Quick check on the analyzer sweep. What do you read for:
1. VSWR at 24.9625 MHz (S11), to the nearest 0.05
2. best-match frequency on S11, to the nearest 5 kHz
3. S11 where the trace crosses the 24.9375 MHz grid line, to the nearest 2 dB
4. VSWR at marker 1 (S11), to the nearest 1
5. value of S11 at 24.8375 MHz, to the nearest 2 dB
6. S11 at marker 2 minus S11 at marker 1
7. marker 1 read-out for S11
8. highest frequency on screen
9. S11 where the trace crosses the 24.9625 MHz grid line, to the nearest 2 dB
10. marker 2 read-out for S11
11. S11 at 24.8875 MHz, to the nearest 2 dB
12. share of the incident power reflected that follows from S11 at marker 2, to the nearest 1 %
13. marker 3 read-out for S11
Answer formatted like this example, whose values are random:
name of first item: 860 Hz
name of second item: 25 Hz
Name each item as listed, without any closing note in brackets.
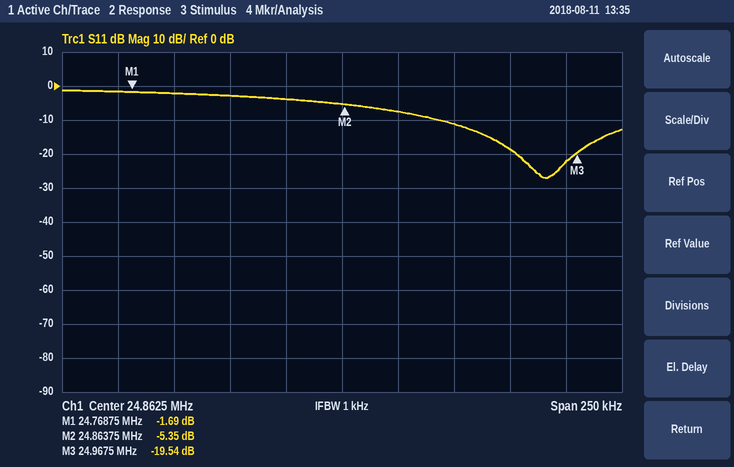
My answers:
VSWR at 24.9625 MHz (S11), to the nearest 0.05: 1.15
best-match frequency on S11, to the nearest 5 kHz: 24.955 MHz
S11 where the trace crosses the 24.9375 MHz grid line, to the nearest 2 dB: -18 dB
VSWR at marker 1 (S11), to the nearest 1: 10
value of S11 at 24.8375 MHz, to the nearest 2 dB: -4 dB
S11 at marker 2 minus S11 at marker 1: -3.66 dB
marker 1 read-out for S11: -1.69 dB
highest frequency on screen: 24.9875 MHz
S11 where the trace crosses the 24.9625 MHz grid line, to the nearest 2 dB: -22 dB
marker 2 read-out for S11: -5.35 dB
S11 at 24.8875 MHz, to the nearest 2 dB: -8 dB
share of the incident power reflected that follows from S11 at marker 2, to the nearest 1 %: 29 %
marker 3 read-out for S11: -19.54 dB
